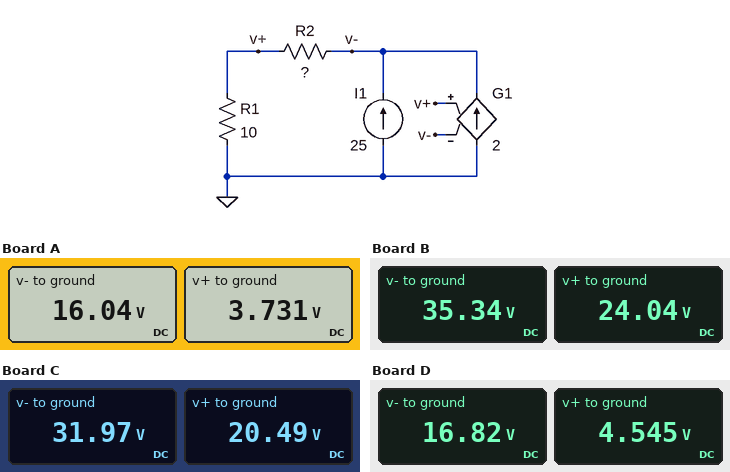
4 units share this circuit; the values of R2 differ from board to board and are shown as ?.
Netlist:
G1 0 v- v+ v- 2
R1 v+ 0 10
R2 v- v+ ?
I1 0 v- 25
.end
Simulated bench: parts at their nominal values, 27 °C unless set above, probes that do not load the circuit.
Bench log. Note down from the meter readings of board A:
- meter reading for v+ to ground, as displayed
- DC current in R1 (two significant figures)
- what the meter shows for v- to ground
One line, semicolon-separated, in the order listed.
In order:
3.731 V; 370 mA; 16.04 V
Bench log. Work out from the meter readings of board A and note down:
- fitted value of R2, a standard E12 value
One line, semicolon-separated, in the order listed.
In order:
33 Ω
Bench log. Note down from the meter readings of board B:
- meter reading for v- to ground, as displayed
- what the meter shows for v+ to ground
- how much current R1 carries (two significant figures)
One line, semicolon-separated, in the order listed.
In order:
35.34 V; 24.04 V; 2.4 A
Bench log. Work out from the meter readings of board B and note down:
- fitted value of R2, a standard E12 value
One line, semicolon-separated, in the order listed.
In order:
4.7 Ω
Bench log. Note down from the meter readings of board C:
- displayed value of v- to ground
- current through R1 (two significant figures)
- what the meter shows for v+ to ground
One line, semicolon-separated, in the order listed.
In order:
31.97 V; 2.0 A; 20.49 V
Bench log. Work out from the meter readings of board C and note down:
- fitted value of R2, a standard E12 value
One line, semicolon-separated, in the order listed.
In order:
5.6 Ω
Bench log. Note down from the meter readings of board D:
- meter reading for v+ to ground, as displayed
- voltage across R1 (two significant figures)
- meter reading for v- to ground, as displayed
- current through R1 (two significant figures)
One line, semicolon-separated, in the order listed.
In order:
4.545 V; 4.5 V; 16.82 V; 450 mA
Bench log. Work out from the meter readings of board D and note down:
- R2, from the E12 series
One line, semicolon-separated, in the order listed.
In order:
27 Ω
